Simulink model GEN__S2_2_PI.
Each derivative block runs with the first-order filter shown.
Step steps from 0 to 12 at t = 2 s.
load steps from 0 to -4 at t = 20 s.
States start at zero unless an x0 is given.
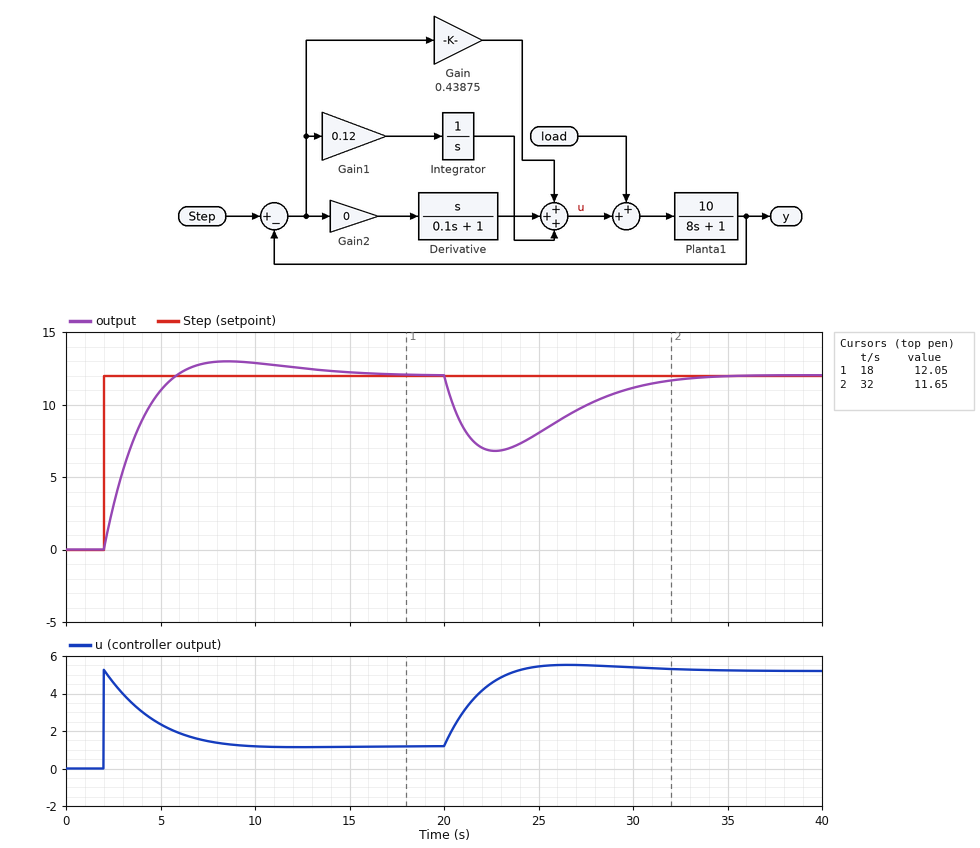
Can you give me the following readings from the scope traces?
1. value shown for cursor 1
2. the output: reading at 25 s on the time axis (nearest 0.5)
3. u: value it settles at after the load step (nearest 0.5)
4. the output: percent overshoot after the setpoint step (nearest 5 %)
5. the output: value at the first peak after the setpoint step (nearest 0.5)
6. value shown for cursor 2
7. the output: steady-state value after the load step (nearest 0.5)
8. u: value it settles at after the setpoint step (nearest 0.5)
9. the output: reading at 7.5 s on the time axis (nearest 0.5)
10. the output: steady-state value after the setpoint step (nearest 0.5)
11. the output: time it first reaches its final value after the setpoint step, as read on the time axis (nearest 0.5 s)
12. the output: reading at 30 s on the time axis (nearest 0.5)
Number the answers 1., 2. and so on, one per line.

1. 12.05
2. 8.0
3. 5.0
4. 10 %
5. 13.0
6. 11.65
7. 12.0
8. 1.0
9. 13.0
10. 12.0
11. 6.0 s
12. 11.0
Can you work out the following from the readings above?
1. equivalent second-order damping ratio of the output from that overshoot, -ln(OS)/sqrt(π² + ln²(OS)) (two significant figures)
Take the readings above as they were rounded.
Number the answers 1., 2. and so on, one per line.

1. 0.59
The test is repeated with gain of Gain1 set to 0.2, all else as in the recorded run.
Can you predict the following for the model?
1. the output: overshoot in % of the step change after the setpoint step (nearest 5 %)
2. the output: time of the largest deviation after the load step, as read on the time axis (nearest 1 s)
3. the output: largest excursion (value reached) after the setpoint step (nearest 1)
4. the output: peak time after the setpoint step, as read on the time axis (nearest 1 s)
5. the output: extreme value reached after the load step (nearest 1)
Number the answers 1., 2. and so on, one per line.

1. 15 %
2. 22 s
3. 14
4. 7 s
5. 7
